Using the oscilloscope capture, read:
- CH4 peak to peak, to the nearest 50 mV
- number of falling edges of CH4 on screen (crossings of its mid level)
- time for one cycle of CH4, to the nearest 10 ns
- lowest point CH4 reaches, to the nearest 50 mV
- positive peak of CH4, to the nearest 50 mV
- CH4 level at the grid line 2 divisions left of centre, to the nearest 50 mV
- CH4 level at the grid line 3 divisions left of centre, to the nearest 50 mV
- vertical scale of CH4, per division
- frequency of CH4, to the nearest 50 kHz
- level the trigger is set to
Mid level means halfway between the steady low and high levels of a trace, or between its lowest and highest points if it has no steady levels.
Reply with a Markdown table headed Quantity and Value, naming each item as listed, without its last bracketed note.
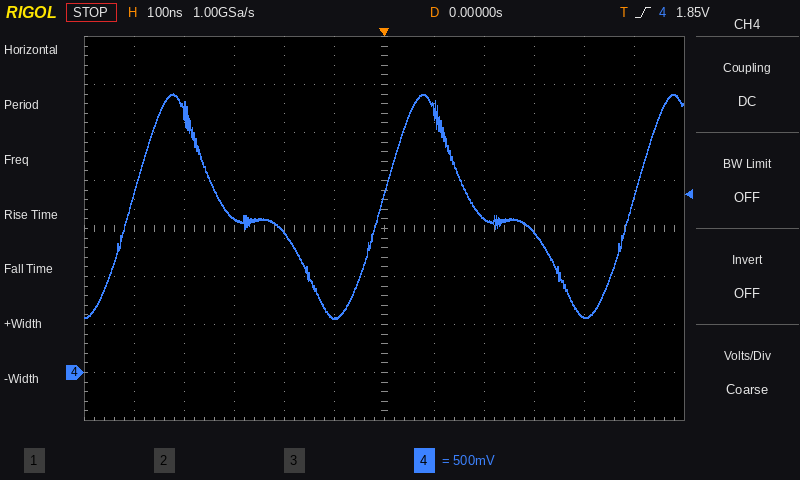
| Quantity | Value |
|---|---|
| CH4 peak to peak, to the nearest 50 mV | 2.35 V |
| number of falling edges of CH4 on screen | 2 |
| time for one cycle of CH4, to the nearest 10 ns | 500 ns |
| lowest point CH4 reaches, to the nearest 50 mV | 550 mV |
| positive peak of CH4, to the nearest 50 mV | 2.90 V |
| CH4 level at the grid line 2 divisions left of centre, to the nearest 50 mV | 1.45 V |
| CH4 level at the grid line 3 divisions left of centre, to the nearest 50 mV | 1.60 V |
| vertical scale of CH4, per division | 500 mV |
| frequency of CH4, to the nearest 50 kHz | 2.00 MHz |
| level the trigger is set to | 1.85 V |
